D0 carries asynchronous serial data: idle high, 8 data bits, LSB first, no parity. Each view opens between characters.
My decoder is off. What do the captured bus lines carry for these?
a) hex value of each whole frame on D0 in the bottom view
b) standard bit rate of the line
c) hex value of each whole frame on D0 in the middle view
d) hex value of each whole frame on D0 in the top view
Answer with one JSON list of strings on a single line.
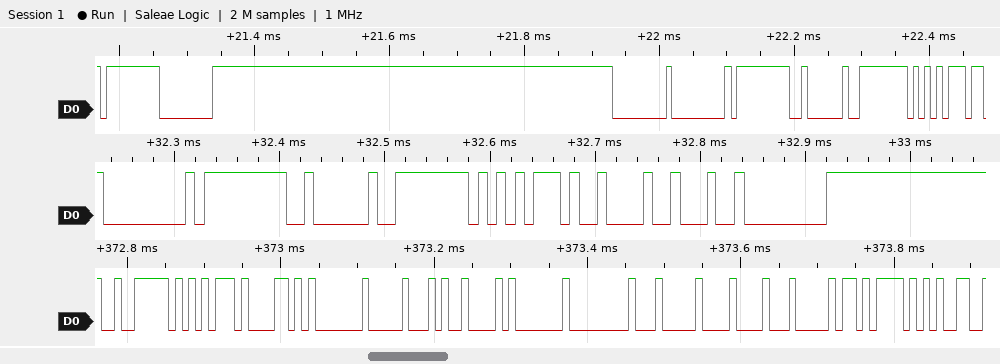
["F2, D5, 61, 01, 10, 09, 01, 00, 04, 08, 04, EB, 95", "115200 baud", "00, FF, 02, FE, D5, 09, 22, 00", "FF, 00, 00, 00, FF, 02, FE, D5"]
